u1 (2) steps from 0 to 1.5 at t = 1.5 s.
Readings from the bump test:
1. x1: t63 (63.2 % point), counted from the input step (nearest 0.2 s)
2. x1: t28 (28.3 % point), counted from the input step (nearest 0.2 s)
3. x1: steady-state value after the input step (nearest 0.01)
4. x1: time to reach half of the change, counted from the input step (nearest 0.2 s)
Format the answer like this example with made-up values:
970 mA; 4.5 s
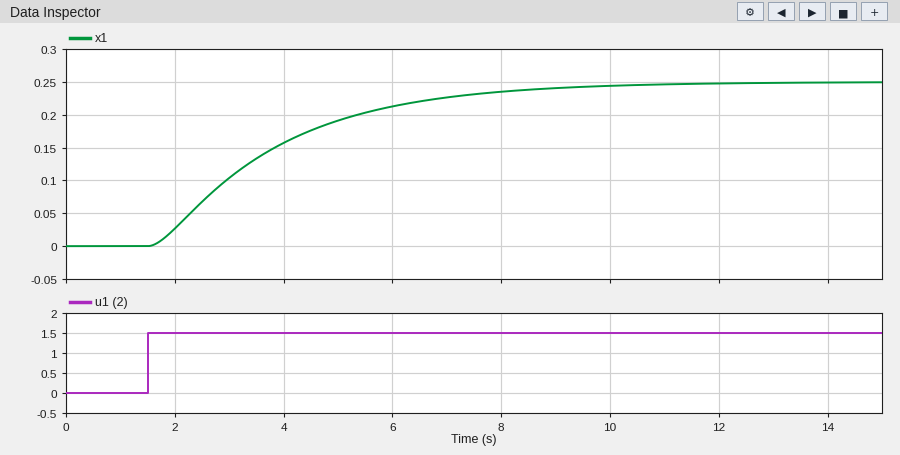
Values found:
2.6 s; 1.0 s; 0.25; 1.8 s
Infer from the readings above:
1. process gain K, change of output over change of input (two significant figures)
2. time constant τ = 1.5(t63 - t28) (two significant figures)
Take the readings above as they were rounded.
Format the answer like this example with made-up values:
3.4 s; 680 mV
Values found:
0.17; 2.4 s
